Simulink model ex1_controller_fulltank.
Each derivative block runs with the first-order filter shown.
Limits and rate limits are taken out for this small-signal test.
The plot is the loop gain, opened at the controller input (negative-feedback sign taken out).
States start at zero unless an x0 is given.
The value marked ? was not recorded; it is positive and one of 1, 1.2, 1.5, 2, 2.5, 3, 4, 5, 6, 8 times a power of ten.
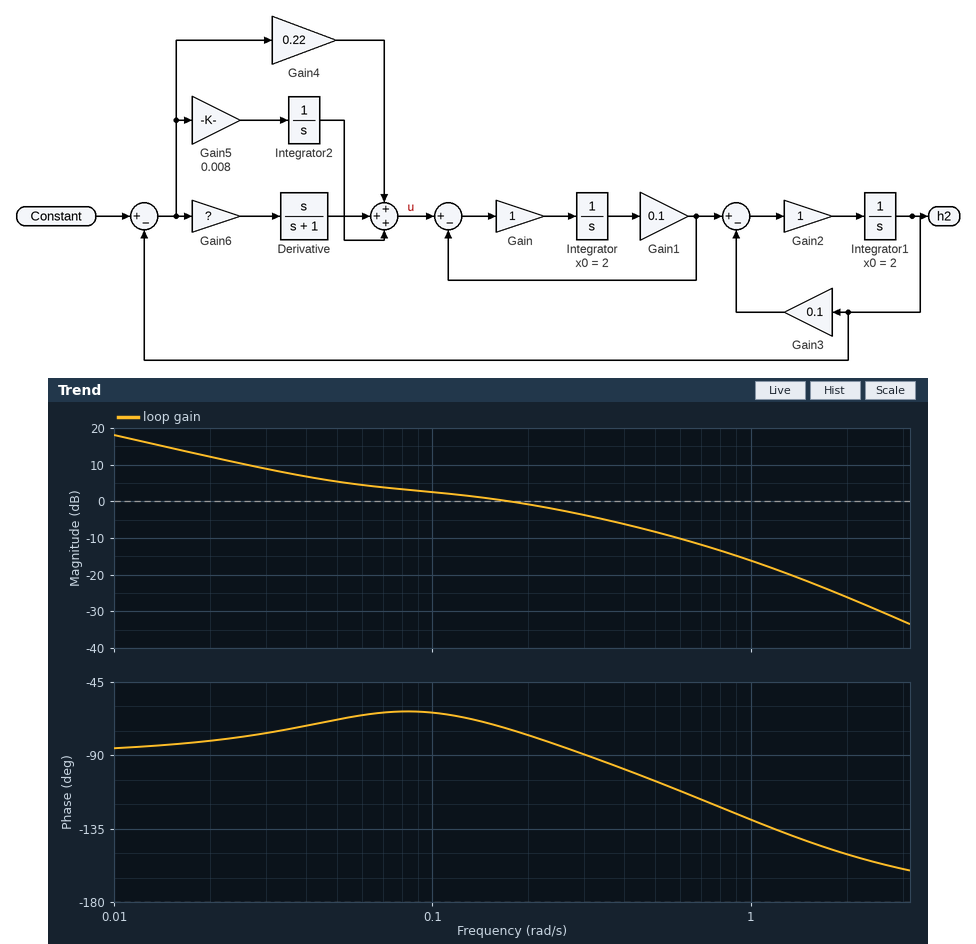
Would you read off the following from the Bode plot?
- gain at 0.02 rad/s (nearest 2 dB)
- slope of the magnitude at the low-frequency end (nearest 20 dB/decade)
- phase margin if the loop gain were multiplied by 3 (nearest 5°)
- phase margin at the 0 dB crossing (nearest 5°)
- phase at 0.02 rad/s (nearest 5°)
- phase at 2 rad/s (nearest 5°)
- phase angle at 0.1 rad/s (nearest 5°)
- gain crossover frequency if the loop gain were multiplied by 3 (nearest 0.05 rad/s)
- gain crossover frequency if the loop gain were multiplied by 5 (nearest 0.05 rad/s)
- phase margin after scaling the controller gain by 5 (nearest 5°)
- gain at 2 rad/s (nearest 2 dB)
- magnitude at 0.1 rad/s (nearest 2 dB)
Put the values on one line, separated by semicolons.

12 dB; -20 dB/decade; 70°; 105°; -80°; -150°; -65°; 0.55 rad/s; 0.85 rad/s; 55°; -26 dB; 2 dB
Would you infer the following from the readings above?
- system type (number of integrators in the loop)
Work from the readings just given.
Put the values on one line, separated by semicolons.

1
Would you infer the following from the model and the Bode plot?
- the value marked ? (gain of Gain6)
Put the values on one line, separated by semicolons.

2
